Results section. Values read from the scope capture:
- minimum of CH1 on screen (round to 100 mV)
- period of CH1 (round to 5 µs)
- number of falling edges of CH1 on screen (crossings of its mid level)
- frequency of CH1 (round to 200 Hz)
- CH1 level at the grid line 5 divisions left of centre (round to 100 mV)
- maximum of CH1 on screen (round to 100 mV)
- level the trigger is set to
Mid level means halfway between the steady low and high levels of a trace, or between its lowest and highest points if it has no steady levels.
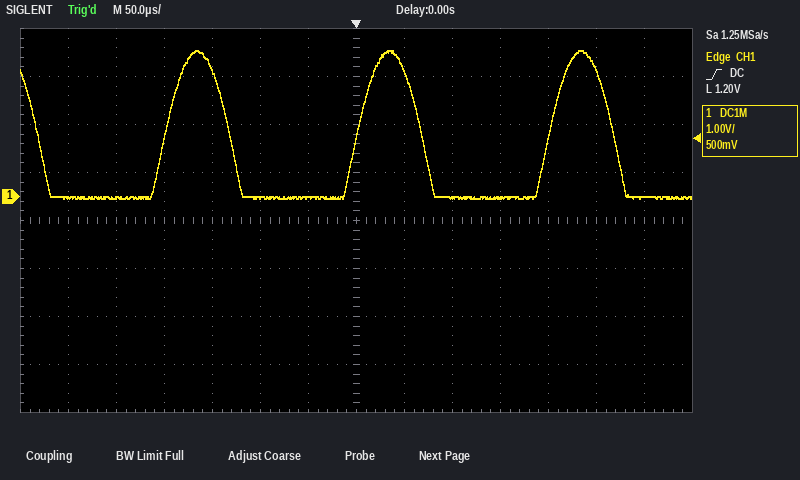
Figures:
0.0 V
200 µs
4
5.0 kHz
0.0 V
3.0 V
1.20 V
